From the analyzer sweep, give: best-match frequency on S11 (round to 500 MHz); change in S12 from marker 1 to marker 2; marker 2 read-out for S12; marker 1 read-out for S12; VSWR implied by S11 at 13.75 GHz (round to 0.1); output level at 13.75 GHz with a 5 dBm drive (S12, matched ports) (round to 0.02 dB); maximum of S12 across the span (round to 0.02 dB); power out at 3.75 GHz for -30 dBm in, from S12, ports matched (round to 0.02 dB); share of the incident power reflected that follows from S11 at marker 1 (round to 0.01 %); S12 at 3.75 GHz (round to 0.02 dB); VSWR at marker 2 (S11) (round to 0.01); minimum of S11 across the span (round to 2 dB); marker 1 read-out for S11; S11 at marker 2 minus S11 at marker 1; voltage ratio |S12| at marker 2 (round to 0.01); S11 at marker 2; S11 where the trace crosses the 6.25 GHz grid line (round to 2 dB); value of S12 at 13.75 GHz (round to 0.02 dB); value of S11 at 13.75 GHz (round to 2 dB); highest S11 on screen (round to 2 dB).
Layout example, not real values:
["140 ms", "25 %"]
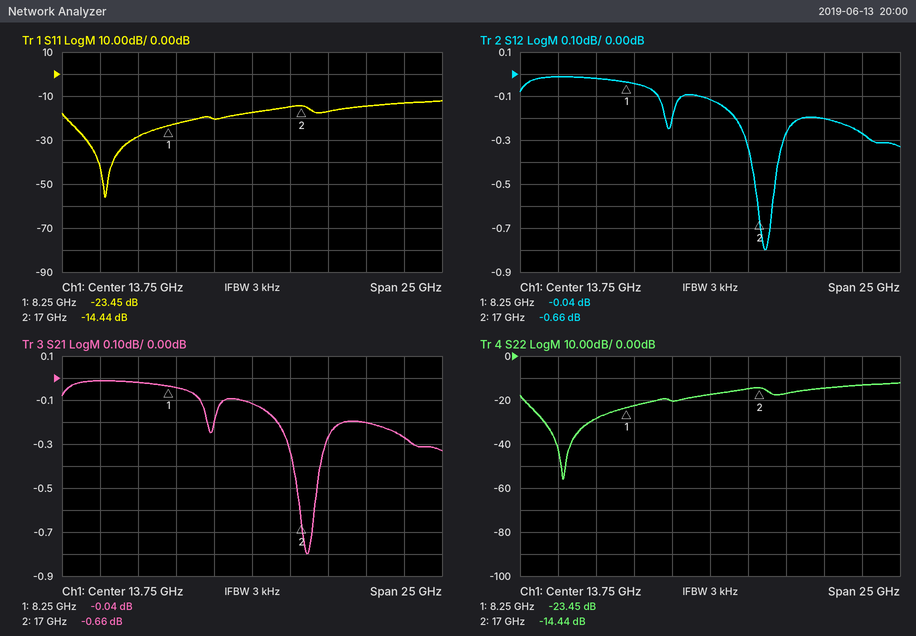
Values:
["4.0 GHz", "-0.62 dB", "-0.66 dB", "-0.04 dB", "1.3", "4.88 dBm", "-0.02 dB", "-30.02 dBm", "0.45 %", "-0.02 dB", "1.47", "-56 dB", "-23.45 dB", "9.01 dB", "0.93", "-14.44 dB", "-28 dB", "-0.12 dB", "-18 dB", "-12 dB"]
